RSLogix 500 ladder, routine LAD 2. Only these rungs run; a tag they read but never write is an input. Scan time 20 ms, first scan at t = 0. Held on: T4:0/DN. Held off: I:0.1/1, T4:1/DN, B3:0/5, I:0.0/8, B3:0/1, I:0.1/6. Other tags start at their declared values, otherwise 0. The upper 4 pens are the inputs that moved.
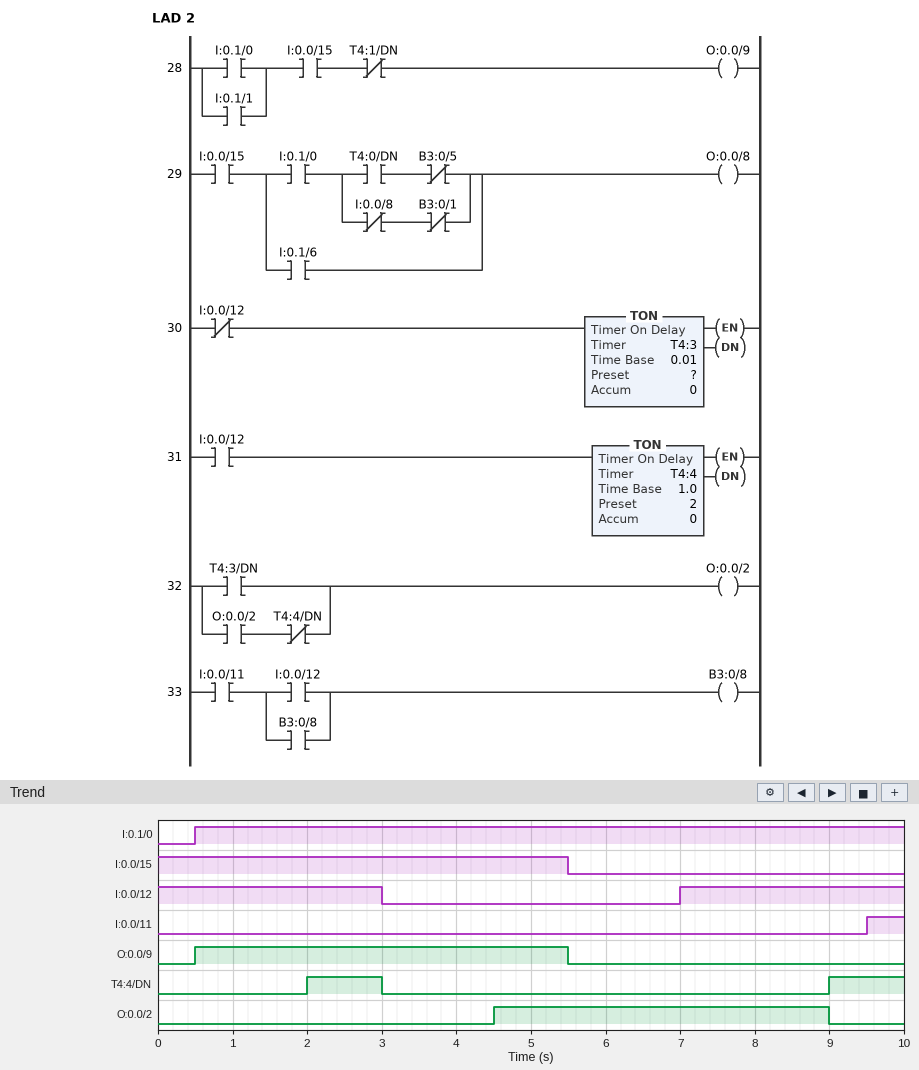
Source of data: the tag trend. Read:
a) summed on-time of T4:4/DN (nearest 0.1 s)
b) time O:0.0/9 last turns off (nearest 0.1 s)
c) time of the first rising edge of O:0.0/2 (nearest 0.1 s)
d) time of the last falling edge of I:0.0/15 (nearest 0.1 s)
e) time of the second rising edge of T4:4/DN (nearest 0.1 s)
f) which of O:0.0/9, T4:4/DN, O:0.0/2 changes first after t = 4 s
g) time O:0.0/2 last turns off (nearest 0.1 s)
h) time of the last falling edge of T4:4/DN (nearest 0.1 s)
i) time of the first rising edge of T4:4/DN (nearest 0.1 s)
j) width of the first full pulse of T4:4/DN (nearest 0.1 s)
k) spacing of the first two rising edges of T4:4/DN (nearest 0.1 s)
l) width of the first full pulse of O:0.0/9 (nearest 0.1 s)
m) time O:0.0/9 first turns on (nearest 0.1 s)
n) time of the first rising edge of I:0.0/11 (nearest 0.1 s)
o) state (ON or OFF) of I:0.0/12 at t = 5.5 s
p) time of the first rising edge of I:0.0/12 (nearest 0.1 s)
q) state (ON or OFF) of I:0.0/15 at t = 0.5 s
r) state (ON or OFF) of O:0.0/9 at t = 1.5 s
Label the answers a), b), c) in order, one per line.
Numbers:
a) 2.0 s
b) 5.5 s
c) 4.5 s
d) 5.5 s
e) 9.0 s
f) O:0.0/2
g) 9.0 s
h) 3.0 s
i) 2.0 s
j) 1.0 s
k) 7.0 s
l) 5.0 s
m) 0.5 s
n) 9.5 s
o) OFF
p) 7.0 s
q) ON
r) ON
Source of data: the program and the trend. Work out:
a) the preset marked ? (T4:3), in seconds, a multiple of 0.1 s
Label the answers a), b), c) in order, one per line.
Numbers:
a) 1.5 s
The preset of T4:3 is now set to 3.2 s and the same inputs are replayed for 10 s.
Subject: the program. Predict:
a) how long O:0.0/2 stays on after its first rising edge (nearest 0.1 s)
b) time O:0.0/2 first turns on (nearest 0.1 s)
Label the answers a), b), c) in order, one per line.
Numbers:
a) 2.8 s
b) 6.2 s
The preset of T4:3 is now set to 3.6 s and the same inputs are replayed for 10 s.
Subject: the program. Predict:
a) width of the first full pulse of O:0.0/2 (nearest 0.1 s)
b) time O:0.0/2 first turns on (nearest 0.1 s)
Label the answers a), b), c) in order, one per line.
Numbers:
a) 2.4 s
b) 6.6 s
